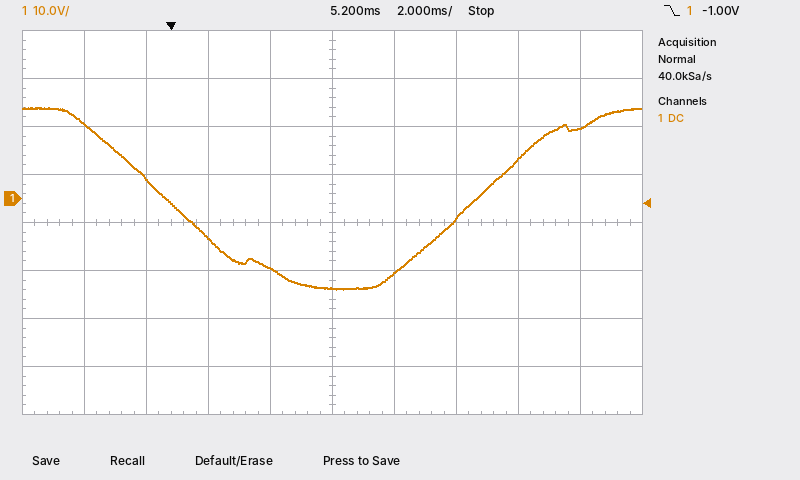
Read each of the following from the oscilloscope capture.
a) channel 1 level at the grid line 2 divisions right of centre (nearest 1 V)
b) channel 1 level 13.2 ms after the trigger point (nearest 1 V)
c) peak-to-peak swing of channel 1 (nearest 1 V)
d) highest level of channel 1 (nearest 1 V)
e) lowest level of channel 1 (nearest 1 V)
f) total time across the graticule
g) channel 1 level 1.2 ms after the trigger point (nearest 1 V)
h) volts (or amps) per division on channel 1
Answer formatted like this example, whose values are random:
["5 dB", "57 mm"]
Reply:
["-4 V", "15 V", "38 V", "19 V", "-19 V", "20 ms", "-8 V", "10 V"]
